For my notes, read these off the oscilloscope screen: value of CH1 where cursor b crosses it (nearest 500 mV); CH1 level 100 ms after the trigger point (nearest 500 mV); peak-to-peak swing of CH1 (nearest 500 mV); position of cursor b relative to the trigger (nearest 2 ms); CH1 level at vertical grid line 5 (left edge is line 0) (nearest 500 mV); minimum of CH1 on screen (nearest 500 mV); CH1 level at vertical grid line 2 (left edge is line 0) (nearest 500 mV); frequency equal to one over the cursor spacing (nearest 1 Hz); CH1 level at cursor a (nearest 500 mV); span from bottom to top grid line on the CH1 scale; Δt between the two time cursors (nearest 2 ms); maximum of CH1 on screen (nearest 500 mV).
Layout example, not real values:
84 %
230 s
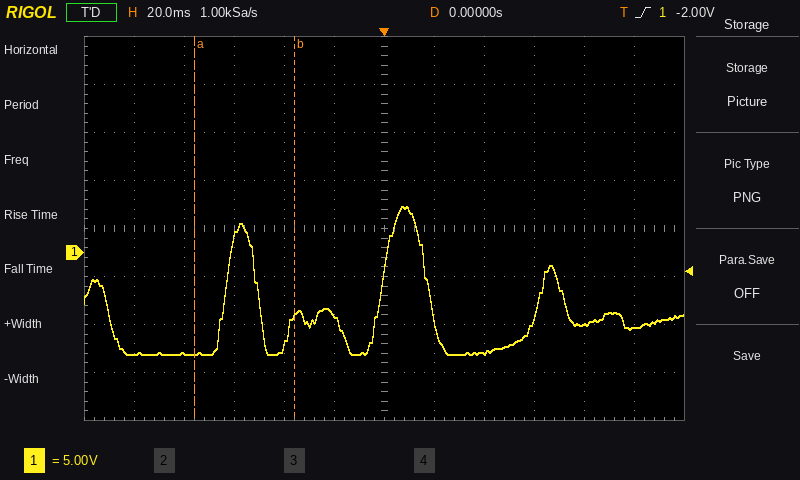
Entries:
-6.5 V
-8.0 V
15.5 V
-36 ms
-6.5 V
-10.5 V
-10.5 V
25 Hz
-10.5 V
40 V
40 ms
5.0 V
